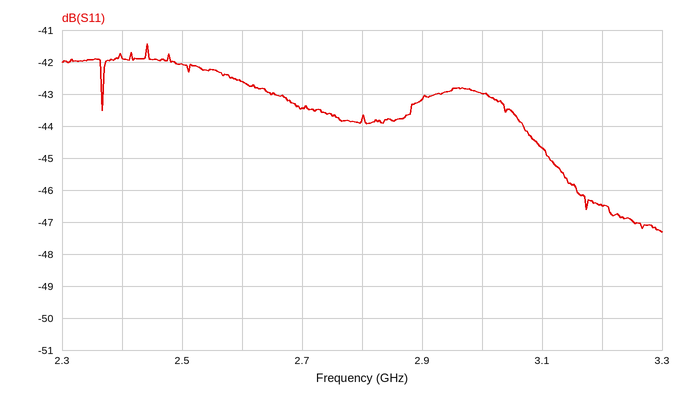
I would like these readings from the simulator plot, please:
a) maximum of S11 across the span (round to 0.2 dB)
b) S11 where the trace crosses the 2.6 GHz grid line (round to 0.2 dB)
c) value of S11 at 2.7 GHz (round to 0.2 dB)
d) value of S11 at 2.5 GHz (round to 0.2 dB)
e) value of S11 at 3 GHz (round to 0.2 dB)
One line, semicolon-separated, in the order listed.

-41.4 dB; -42.6 dB; -43.4 dB; -42.0 dB; -43.0 dB
